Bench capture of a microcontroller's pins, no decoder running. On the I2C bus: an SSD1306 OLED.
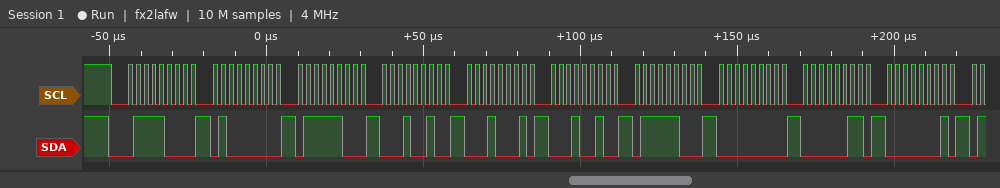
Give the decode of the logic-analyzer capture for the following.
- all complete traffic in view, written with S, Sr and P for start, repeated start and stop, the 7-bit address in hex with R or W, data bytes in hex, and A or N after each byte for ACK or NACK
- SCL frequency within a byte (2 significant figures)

S 3CW A 40 A 7C A 12 A 11 A 12 A 7C A 00 A 03 A 01 A
400 kHz
